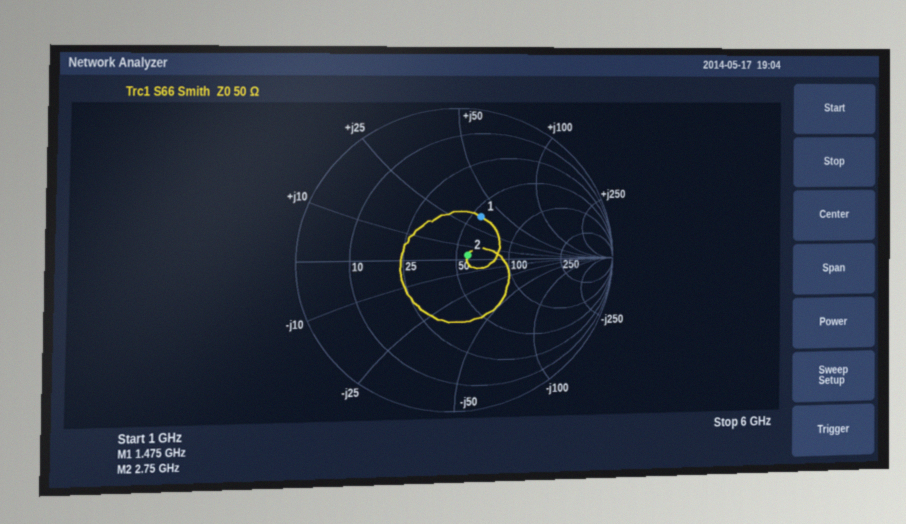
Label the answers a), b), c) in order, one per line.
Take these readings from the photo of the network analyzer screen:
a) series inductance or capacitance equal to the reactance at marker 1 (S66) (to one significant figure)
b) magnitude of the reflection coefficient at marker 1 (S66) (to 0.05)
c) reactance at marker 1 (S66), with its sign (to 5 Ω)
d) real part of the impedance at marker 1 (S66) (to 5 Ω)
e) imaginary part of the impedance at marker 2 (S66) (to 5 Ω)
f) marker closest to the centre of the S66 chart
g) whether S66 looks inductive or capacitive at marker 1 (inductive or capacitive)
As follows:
a) 4 nH
b) 0.30
c) +35 Ω
d) 55 Ω
e) +5 Ω
f) marker 2
g) inductive
